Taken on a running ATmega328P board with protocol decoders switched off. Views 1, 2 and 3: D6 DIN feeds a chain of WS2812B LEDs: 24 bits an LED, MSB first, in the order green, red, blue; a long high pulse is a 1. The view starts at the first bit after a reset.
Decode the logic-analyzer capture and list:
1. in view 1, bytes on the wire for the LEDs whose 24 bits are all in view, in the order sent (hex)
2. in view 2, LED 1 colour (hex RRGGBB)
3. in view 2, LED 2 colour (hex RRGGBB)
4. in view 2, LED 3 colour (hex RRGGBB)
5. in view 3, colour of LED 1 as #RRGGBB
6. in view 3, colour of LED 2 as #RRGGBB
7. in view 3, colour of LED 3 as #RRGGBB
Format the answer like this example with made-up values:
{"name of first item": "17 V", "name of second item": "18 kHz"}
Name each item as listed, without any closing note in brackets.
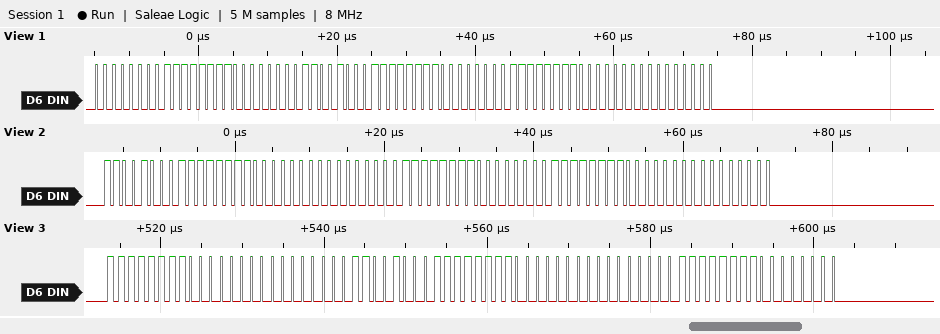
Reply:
{"in view 1, bytes on the wire for the LEDs whose 24 bits are all in view, in the order sent": "00 FF 00 C8 FF 00 FF 00 00", "in view 2, LED 1 colour": "#FFC800", "in view 2, LED 2 colour": "#FF0000", "in view 2, LED 3 colour": "#00FF00", "in view 3, colour of LED 1 as #RRGGBB": "#00FF00", "in view 3, colour of LED 2 as #RRGGBB": "#FFC800", "in view 3, colour of LED 3 as #RRGGBB": "#FF0000"}
